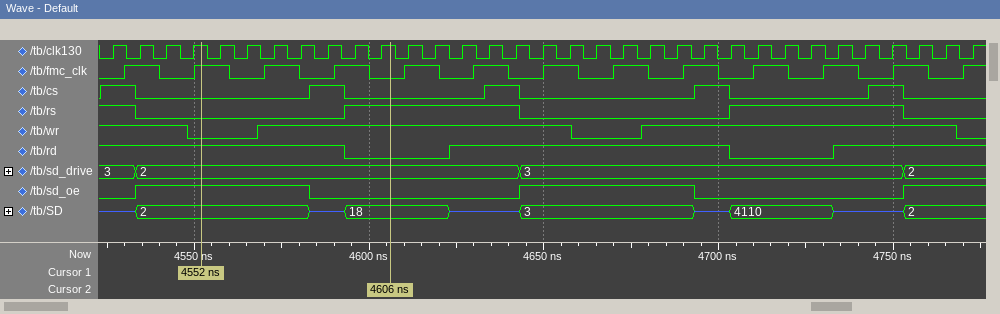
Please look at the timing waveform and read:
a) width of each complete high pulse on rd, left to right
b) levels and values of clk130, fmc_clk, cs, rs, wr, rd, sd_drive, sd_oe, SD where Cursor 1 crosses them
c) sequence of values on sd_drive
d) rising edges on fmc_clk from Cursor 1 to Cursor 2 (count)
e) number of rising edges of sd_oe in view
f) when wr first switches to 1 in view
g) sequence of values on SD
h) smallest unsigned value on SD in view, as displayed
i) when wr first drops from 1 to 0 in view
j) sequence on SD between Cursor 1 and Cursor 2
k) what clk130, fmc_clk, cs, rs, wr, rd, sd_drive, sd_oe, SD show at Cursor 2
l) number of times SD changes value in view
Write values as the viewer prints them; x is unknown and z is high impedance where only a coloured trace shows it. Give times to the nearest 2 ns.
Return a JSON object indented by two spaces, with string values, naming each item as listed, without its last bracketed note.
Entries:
{
  "width of each complete high pulse on rd, left to right": "80 ns",
  "levels and values of clk130, fmc_clk, cs, rs, wr, rd, sd_drive, sd_oe, SD where Cursor 1 crosses them": "clk130=1, fmc_clk=1, cs=0, rs=0, wr=0, rd=1, sd_drive=2, sd_oe=1, SD=2",
  "sequence of values on sd_drive": "3, 2, 3, 2",
  "rising edges on fmc_clk from Cursor 1 to Cursor 2": "2",
  "number of rising edges of sd_oe in view": "3",
  "when wr first switches to 1 in view": "4568 ns",
  "sequence of values on SD": "z, 2, z, 18, z, 3, z, 4110, z, 2",
  "smallest unsigned value on SD in view, as displayed": "2",
  "when wr first drops from 1 to 0 in view": "4548 ns",
  "sequence on SD between Cursor 1 and Cursor 2": "2, z, 18",
  "what clk130, fmc_clk, cs, rs, wr, rd, sd_drive, sd_oe, SD show at Cursor 2": "clk130=1, fmc_clk=0, cs=0, rs=1, wr=1, rd=0, sd_drive=2, sd_oe=0, SD=18",
  "number of times SD changes value in view": "9"
}
